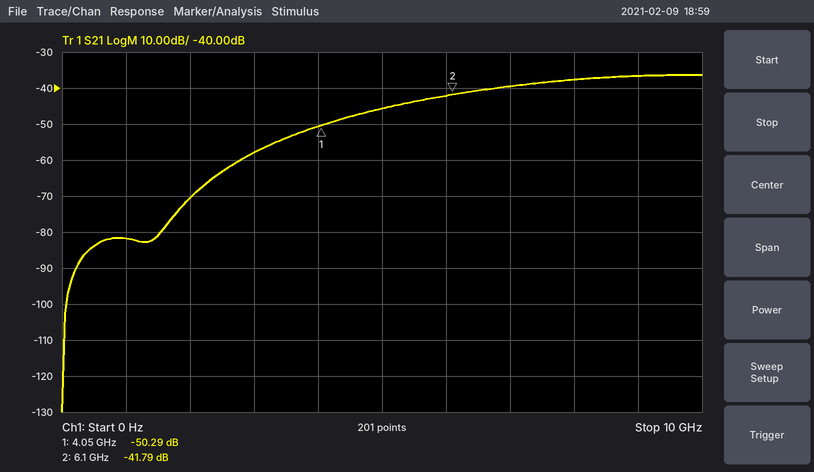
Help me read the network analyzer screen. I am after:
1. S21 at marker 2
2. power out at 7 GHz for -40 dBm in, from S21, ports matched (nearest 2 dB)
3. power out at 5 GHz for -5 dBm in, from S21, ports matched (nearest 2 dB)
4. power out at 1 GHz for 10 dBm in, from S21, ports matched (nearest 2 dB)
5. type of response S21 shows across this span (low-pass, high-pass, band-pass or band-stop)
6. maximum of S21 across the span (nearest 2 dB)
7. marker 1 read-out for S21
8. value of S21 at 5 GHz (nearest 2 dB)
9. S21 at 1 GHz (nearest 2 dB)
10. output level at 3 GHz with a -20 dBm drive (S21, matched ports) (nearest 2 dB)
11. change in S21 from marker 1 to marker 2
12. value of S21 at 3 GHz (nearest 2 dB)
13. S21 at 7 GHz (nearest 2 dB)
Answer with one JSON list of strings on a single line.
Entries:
["-41.79 dB", "-80 dBm", "-50 dBm", "-72 dBm", "high-pass", "-36 dB", "-50.29 dB", "-46 dB", "-82 dB", "-78 dBm", "8.50 dB", "-58 dB", "-40 dB"]
